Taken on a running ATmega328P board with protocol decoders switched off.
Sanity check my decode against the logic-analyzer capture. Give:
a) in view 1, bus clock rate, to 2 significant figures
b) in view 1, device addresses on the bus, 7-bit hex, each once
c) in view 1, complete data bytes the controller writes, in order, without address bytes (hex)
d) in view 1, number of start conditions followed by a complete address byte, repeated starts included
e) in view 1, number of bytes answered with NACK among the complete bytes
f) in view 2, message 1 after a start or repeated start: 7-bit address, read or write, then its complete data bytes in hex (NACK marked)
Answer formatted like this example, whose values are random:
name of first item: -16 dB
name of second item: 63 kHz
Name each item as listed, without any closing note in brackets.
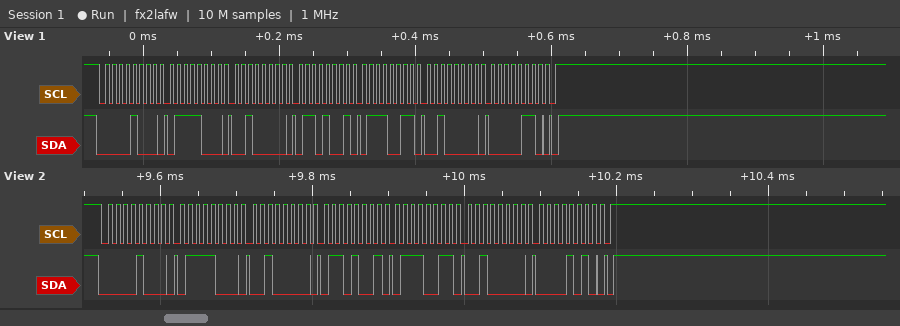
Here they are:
in view 1, bus clock rate, to 2 significant figures: 100 kHz
in view 1, device addresses on the bus, 7-bit hex, each once: 0x04
in view 1, complete data bytes the controller writes, in order, without address bytes: 78 20 69 73 20 06
in view 1, number of start conditions followed by a complete address byte, repeated starts included: 1
in view 1, number of bytes answered with NACK among the complete bytes: 0
in view 2, message 1 after a start or repeated start: 7-bit address, read or write, then its complete data bytes in hex: 0x04 write: 78 20 69 73 20 0A
